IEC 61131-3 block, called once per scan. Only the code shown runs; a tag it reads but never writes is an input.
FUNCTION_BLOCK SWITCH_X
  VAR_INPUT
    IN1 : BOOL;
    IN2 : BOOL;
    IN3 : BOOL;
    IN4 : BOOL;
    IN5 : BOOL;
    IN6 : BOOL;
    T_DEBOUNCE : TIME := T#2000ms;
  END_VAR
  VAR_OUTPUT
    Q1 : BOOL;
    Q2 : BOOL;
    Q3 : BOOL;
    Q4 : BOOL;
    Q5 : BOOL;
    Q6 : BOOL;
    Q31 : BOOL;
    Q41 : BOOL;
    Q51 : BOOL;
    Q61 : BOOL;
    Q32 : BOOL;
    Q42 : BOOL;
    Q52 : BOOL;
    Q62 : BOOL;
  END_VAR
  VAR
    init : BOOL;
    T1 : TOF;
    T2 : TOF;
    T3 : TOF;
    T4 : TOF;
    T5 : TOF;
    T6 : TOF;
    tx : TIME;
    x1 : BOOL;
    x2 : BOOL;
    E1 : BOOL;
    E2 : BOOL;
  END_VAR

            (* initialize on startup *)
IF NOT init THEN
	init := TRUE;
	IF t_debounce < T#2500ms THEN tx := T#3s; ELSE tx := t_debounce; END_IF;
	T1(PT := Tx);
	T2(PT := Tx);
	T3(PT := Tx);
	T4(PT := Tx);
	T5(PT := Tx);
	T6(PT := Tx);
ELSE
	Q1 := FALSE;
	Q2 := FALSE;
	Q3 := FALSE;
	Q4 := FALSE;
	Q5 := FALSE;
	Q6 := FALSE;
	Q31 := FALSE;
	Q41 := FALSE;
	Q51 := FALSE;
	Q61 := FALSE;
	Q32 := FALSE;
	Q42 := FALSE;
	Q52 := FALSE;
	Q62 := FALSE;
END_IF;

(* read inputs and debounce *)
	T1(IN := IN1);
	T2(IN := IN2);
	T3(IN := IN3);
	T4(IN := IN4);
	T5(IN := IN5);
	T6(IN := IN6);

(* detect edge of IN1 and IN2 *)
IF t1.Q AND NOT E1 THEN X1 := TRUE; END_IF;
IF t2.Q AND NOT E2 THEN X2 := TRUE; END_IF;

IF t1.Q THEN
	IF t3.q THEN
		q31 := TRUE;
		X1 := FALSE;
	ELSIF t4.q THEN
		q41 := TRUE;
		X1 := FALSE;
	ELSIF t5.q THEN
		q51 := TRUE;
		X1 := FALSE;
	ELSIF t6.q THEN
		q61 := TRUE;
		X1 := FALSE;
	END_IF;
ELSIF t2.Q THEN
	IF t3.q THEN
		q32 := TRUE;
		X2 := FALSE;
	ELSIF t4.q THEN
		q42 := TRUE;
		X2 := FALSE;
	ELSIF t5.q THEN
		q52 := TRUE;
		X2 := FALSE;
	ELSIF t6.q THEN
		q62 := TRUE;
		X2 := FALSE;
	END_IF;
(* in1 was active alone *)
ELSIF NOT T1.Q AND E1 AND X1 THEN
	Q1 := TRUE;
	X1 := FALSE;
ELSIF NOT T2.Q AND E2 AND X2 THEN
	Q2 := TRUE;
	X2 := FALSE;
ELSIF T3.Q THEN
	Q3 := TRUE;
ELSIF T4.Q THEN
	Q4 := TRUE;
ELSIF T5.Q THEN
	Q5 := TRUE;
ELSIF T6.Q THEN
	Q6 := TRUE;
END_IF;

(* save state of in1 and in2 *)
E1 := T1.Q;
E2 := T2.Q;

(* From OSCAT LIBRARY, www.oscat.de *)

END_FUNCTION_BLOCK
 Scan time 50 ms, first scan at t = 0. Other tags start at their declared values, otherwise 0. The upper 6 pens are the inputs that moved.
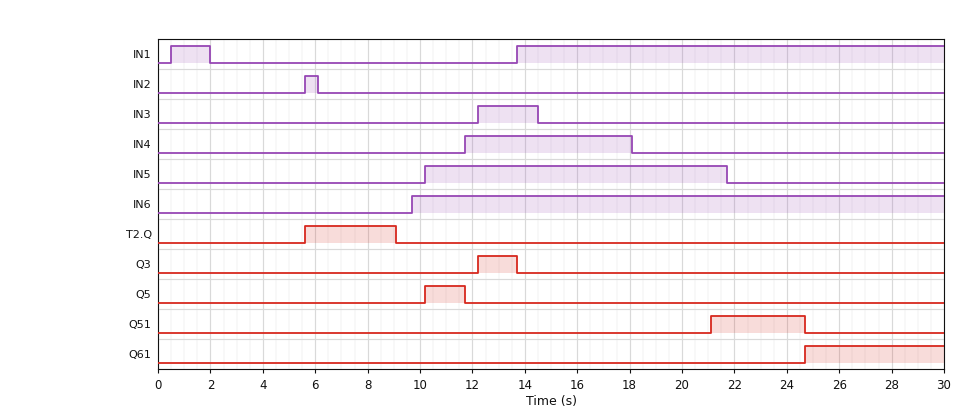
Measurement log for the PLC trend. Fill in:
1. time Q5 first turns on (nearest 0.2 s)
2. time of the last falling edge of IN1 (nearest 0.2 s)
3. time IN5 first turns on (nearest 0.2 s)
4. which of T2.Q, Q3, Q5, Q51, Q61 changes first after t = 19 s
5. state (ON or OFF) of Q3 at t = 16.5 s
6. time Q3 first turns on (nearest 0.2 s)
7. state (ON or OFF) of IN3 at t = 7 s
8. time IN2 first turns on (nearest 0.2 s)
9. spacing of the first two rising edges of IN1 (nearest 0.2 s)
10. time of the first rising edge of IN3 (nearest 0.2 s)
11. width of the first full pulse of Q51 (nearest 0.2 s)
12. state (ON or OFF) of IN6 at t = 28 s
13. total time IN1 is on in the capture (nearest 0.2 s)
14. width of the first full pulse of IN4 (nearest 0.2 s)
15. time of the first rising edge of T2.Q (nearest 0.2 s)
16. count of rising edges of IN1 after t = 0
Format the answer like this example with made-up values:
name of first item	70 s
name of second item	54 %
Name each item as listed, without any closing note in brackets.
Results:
time Q5 first turns on	10.2 s
time of the last falling edge of IN1	2.0 s
time IN5 first turns on	10.2 s
which of T2.Q, Q3, Q5, Q51, Q61 changes first after t = 19 s	Q51
state (ON or OFF) of Q3 at t = 16.5 s	OFF
time Q3 first turns on	12.2 s
state (ON or OFF) of IN3 at t = 7 s	OFF
time IN2 first turns on	5.6 s
spacing of the first two rising edges of IN1	13.2 s
time of the first rising edge of IN3	12.2 s
width of the first full pulse of Q51	3.6 s
state (ON or OFF) of IN6 at t = 28 s	ON
total time IN1 is on in the capture	17.8 s
width of the first full pulse of IN4	6.4 s
time of the first rising edge of T2.Q	5.6 s
count of rising edges of IN1 after t = 0	2
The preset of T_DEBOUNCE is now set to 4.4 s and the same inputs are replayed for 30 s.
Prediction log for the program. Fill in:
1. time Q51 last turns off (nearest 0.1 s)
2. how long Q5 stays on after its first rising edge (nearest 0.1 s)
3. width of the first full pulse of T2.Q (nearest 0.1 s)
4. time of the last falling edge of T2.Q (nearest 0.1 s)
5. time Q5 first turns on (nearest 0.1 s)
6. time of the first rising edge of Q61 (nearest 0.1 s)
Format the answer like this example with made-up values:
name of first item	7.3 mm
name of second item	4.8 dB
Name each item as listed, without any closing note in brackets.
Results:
time Q51 last turns off	26.1 s
how long Q5 stays on after its first rising edge	1.2 s
width of the first full pulse of T2.Q	4.9 s
time of the last falling edge of T2.Q	10.5 s
time Q5 first turns on	10.5 s
time of the first rising edge of Q61	26.1 s
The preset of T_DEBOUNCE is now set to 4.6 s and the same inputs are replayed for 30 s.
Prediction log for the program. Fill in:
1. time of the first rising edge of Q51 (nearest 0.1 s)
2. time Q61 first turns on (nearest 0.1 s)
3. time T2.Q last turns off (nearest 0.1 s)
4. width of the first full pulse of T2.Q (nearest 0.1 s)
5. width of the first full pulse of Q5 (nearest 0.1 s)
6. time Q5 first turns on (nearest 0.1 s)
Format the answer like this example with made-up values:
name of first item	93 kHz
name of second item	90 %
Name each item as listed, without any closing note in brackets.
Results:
time of the first rising edge of Q51	22.7 s
time Q61 first turns on	26.3 s
time T2.Q last turns off	10.7 s
width of the first full pulse of T2.Q	5.1 s
width of the first full pulse of Q5	1.0 s
time Q5 first turns on	10.7 s
